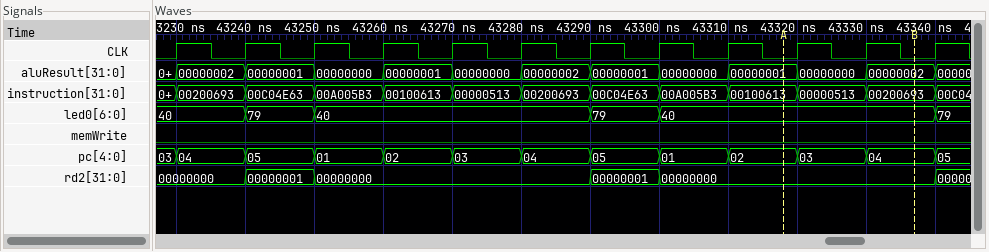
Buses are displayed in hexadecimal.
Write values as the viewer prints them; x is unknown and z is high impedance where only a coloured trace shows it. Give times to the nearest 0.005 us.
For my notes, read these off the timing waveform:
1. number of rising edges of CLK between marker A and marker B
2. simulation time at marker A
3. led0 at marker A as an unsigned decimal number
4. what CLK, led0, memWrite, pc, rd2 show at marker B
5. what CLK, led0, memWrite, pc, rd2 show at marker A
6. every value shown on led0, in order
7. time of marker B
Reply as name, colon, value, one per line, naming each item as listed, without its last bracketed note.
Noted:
number of rising edges of CLK between marker A and marker B: 2
simulation time at marker A: 43.32 us
led0 at marker A as an unsigned decimal number: 64
what CLK, led0, memWrite, pc, rd2 show at marker B: CLK=0, led0=40, memWrite=0, pc=04, rd2=00000000
what CLK, led0, memWrite, pc, rd2 show at marker A: CLK=0, led0=40, memWrite=0, pc=02, rd2=00000000
every value shown on led0, in order: 40, 79, 40, 79, 40, 79
time of marker B: 43.335 us
